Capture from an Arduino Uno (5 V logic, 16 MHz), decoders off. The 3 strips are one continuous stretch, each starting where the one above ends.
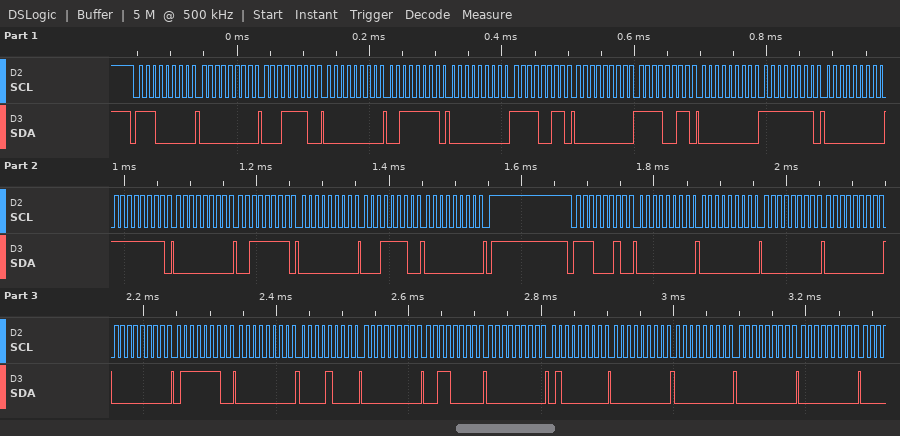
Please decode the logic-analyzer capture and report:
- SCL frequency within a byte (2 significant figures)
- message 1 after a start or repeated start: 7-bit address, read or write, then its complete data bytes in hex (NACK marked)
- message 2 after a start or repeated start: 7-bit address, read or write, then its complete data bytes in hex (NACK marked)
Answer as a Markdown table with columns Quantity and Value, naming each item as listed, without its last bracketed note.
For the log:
| Quantity | Value |
|---|---|
| SCL frequency within a byte | 100 kHz |
| message 1 after a start or repeated start: 7-bit address, read or write, then its complete data bytes in hex | 0x70 write: 00 1E 00 3F 00 F3 00 F3 00 FF 00 FF 00 3F 00 1E 00 |
| message 2 after a start or repeated start: 7-bit address, read or write, then its complete data bytes in hex | 0x71 write: 00 00 00 00 00 7E 00 08 00 30 00 40 00 00 00 00 |
